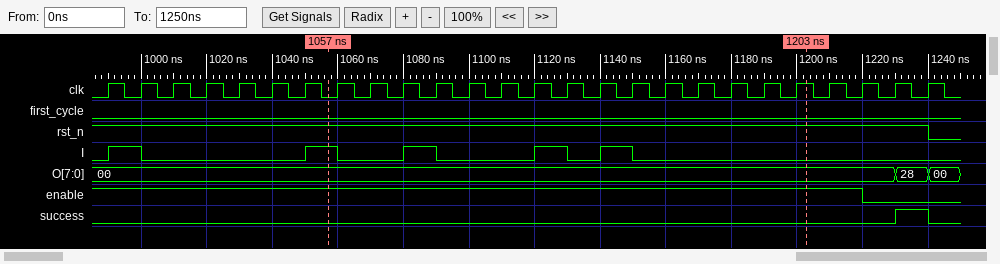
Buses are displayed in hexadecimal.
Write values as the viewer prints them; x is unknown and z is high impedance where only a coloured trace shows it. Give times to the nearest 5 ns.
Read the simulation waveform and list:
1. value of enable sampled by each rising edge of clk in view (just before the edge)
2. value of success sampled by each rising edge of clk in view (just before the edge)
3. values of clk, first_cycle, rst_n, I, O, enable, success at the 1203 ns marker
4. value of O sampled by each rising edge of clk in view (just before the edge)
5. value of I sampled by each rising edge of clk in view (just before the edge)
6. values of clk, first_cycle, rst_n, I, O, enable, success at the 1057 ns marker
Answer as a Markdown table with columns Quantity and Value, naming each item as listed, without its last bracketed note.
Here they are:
| Quantity | Value |
|---|---|
| value of enable sampled by each rising edge of clk in view | 1 1 1 1 1 1 1 1 1 1 1 1 1 1 1 1 1 1 1 1 1 1 1 1 0 0 |
| value of success sampled by each rising edge of clk in view | 0 0 0 0 0 0 0 0 0 0 0 0 0 0 0 0 0 0 0 0 0 0 0 0 0 1 |
| values of clk, first_cycle, rst_n, I, O, enable, success at the 1203 ns marker | clk=1, first_cycle=0, rst_n=1, I=0, O=00, enable=1, success=0 |
| value of O sampled by each rising edge of clk in view | 00, 00, 00, 00, 00, 00, 00, 00, 00, 00, 00, 00, 00, 00, 00, 00, 00, 00, 00, 00, 00, 00, 00, 00, 00, 28 |
| value of I sampled by each rising edge of clk in view | 0 1 0 0 0 0 0 1 0 0 1 0 0 0 1 0 1 0 0 0 0 0 0 0 0 0 |
| values of clk, first_cycle, rst_n, I, O, enable, success at the 1057 ns marker | clk=0, first_cycle=0, rst_n=1, I=1, O=00, enable=1, success=0 |
